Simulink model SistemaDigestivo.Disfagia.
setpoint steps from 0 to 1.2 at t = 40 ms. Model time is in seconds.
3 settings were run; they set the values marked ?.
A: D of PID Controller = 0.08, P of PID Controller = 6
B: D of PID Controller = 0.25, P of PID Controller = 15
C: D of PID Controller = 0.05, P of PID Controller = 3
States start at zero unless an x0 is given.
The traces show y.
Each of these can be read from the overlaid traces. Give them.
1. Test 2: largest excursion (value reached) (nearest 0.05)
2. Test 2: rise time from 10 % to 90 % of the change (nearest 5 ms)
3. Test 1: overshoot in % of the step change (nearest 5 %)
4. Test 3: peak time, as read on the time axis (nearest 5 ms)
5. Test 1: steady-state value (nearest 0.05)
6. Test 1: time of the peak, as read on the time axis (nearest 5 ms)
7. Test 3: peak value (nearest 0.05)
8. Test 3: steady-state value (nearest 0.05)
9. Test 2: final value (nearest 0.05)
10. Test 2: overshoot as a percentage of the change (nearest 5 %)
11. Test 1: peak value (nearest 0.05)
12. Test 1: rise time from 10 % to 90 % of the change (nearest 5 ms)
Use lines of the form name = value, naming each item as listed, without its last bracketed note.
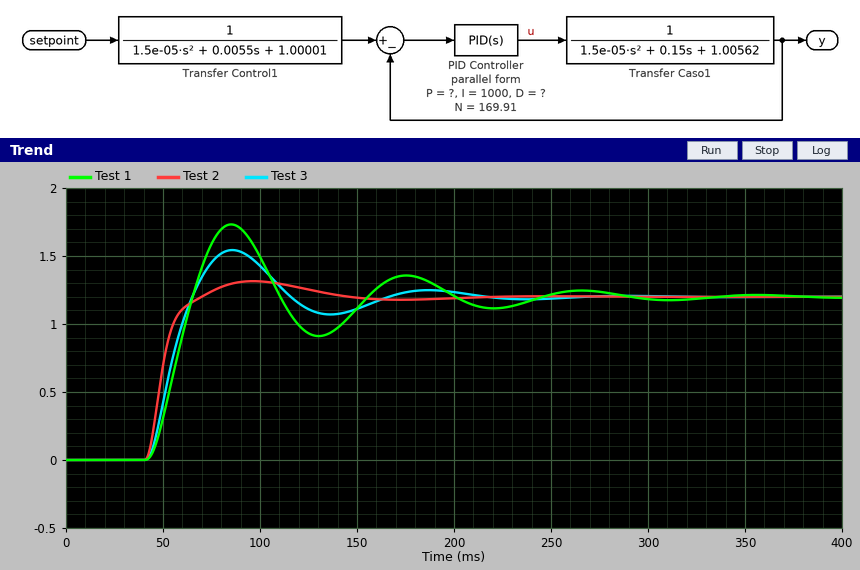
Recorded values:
Test 2: largest excursion (value reached) = 1.30
Test 2: rise time from 10 % to 90 % of the change = 15 ms
Test 1: overshoot in % of the step change = 45 %
Test 3: peak time, as read on the time axis = 85 ms
Test 1: steady-state value = 1.20
Test 1: time of the peak, as read on the time axis = 85 ms
Test 3: peak value = 1.55
Test 3: steady-state value = 1.20
Test 2: final value = 1.20
Test 2: overshoot as a percentage of the change = 10 %
Test 1: peak value = 1.75
Test 1: rise time from 10 % to 90 % of the change = 15 ms
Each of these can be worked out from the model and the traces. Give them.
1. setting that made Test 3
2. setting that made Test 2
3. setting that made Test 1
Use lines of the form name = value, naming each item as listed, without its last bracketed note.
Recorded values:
setting that made Test 3 = A
setting that made Test 2 = B
setting that made Test 1 = C
